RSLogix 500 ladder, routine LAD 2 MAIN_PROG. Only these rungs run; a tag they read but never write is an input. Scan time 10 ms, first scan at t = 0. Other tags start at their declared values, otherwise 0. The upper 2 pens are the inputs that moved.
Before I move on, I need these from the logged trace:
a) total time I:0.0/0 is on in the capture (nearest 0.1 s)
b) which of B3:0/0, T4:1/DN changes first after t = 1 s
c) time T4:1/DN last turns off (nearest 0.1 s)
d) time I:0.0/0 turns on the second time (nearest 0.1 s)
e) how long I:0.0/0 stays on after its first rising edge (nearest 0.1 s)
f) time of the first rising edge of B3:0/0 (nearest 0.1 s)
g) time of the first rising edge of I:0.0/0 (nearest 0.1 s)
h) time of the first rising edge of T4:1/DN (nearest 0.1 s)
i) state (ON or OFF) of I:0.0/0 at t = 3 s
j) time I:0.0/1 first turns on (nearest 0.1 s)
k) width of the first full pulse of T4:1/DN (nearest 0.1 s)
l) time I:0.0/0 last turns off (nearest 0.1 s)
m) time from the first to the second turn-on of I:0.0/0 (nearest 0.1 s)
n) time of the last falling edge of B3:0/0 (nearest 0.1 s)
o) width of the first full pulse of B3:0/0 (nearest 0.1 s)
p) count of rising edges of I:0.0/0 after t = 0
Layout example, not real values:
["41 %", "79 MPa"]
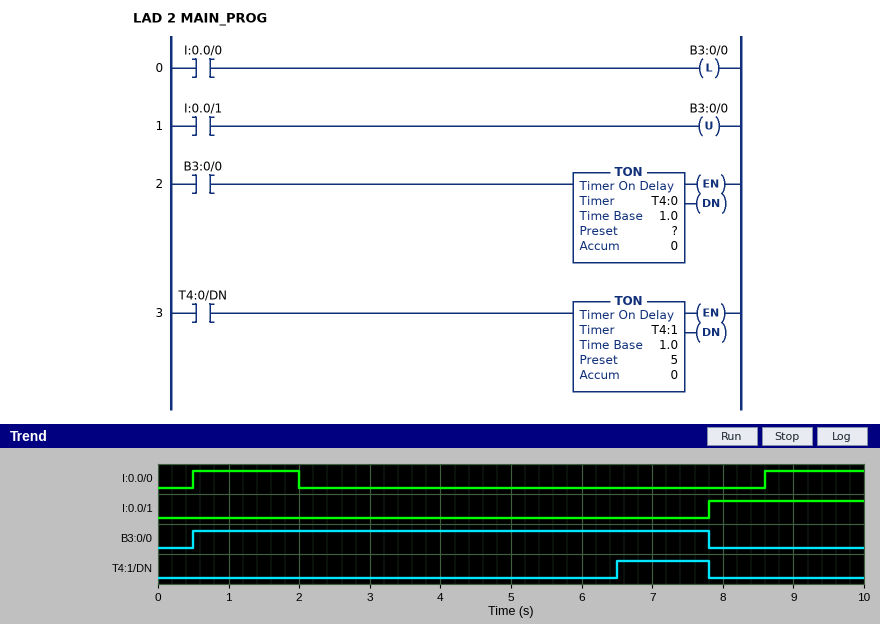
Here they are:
["2.9 s", "T4:1/DN", "7.8 s", "8.6 s", "1.5 s", "0.5 s", "0.5 s", "6.5 s", "OFF", "7.8 s", "1.3 s", "2.0 s", "8.1 s", "7.8 s", "7.3 s", "2"]
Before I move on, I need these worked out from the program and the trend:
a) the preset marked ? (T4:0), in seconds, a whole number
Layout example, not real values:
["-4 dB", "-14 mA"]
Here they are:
["1 s"]
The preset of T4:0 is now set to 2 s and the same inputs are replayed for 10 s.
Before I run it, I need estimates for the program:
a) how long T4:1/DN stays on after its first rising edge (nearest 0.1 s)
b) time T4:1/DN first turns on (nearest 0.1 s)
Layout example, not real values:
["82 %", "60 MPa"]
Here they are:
["0.3 s", "7.5 s"]
